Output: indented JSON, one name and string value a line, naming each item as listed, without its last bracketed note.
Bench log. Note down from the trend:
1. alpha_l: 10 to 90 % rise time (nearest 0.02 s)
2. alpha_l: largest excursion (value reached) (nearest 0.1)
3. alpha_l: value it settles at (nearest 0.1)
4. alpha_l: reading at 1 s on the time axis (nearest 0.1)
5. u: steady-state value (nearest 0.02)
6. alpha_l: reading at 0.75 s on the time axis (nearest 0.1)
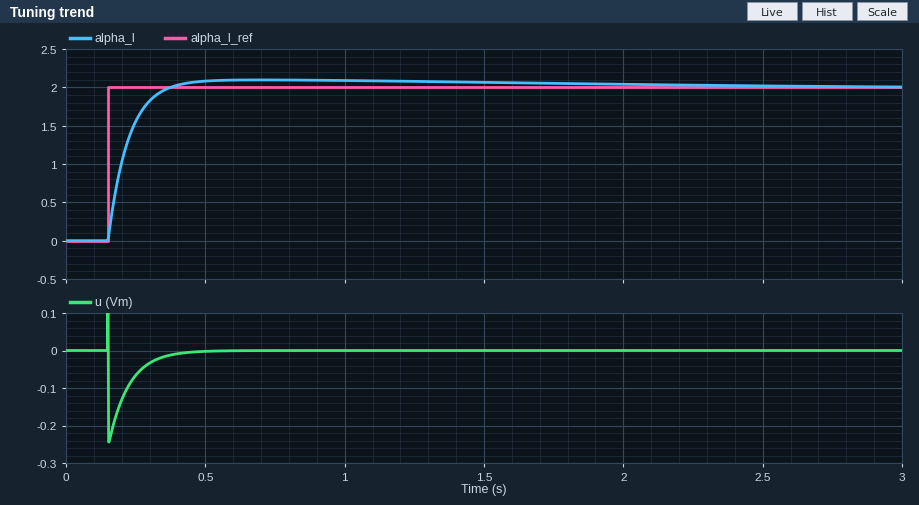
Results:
{
  "alpha_l: 10 to 90 % rise time": "0.14 s",
  "alpha_l: largest excursion (value reached)": "2.1",
  "alpha_l: value it settles at": "2.0",
  "alpha_l: reading at 1 s on the time axis": "2.1",
  "u: steady-state value": "0.00",
  "alpha_l: reading at 0.75 s on the time axis": "2.1"
}
